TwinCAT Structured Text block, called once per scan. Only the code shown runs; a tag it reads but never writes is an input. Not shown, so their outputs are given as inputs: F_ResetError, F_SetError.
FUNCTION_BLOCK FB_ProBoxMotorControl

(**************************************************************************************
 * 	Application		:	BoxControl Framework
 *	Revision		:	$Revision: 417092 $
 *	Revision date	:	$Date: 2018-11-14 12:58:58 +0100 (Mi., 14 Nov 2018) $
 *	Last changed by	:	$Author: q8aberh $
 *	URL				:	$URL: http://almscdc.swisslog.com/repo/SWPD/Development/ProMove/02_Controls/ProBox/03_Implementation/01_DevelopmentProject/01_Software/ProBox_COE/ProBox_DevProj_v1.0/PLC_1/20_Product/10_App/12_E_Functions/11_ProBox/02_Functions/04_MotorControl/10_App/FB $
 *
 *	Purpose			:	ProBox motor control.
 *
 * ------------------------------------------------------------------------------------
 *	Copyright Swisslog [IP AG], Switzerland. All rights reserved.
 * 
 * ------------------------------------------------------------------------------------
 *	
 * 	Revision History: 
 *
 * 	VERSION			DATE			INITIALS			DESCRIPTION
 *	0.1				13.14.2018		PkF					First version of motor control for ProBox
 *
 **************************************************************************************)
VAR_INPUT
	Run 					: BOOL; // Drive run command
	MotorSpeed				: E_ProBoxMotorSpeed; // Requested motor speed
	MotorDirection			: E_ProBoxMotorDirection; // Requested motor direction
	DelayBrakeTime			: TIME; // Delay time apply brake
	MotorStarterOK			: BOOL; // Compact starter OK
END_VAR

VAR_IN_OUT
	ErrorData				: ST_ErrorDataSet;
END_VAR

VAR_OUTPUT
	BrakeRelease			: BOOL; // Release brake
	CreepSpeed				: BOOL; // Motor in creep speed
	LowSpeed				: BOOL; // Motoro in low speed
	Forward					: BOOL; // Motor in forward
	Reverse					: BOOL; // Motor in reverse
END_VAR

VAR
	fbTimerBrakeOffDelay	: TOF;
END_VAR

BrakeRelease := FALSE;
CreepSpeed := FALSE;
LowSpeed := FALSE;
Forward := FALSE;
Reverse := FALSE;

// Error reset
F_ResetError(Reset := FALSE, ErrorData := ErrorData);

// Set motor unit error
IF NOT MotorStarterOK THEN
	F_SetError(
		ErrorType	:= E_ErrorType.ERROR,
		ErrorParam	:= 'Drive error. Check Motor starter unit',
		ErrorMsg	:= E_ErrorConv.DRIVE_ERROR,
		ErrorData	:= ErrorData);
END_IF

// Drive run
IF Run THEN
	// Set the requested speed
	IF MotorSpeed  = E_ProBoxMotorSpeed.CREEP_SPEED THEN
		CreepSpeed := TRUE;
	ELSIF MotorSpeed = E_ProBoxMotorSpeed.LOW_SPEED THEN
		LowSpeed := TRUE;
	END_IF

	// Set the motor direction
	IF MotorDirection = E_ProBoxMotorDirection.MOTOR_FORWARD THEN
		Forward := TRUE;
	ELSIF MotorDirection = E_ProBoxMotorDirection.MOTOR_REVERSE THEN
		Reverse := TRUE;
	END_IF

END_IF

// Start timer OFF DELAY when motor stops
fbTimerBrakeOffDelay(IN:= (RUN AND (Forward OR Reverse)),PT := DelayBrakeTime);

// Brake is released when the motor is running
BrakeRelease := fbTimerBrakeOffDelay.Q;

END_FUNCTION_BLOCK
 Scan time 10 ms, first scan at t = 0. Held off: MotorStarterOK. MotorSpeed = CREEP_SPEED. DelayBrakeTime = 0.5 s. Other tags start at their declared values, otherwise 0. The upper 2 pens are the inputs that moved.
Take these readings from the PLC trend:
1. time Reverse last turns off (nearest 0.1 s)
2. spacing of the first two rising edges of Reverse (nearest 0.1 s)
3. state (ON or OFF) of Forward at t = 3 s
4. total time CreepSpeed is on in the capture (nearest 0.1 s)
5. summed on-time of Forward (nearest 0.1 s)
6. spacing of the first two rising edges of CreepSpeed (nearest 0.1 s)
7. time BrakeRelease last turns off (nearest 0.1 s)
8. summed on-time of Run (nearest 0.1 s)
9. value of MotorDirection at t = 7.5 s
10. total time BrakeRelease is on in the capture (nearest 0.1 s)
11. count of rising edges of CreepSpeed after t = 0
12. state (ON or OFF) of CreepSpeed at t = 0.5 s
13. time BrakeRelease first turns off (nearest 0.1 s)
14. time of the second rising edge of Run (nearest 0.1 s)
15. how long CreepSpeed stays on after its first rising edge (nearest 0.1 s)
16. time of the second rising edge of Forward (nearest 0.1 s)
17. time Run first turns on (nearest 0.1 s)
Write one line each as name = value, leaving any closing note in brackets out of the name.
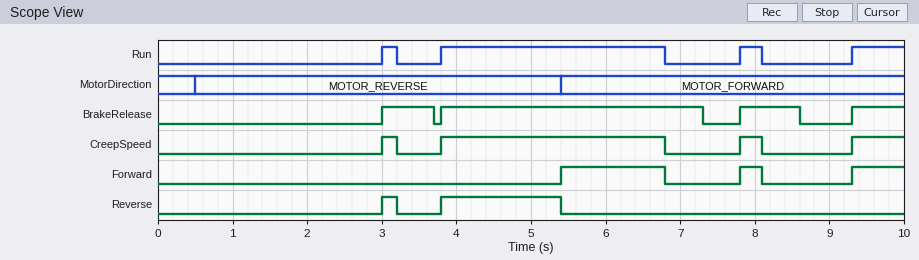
time Reverse last turns off = 5.4 s
spacing of the first two rising edges of Reverse = 0.8 s
state (ON or OFF) of Forward at t = 3 s = OFF
total time CreepSpeed is on in the capture = 4.2 s
summed on-time of Forward = 2.4 s
spacing of the first two rising edges of CreepSpeed = 0.8 s
time BrakeRelease last turns off = 8.6 s
summed on-time of Run = 4.2 s
value of MotorDirection at t = 7.5 s = MOTOR_FORWARD
total time BrakeRelease is on in the capture = 5.7 s
count of rising edges of CreepSpeed after t = 0 = 4
state (ON or OFF) of CreepSpeed at t = 0.5 s = OFF
time BrakeRelease first turns off = 3.7 s
time of the second rising edge of Run = 3.8 s
how long CreepSpeed stays on after its first rising edge = 0.2 s
time of the second rising edge of Forward = 7.8 s
time Run first turns on = 3.0 s
